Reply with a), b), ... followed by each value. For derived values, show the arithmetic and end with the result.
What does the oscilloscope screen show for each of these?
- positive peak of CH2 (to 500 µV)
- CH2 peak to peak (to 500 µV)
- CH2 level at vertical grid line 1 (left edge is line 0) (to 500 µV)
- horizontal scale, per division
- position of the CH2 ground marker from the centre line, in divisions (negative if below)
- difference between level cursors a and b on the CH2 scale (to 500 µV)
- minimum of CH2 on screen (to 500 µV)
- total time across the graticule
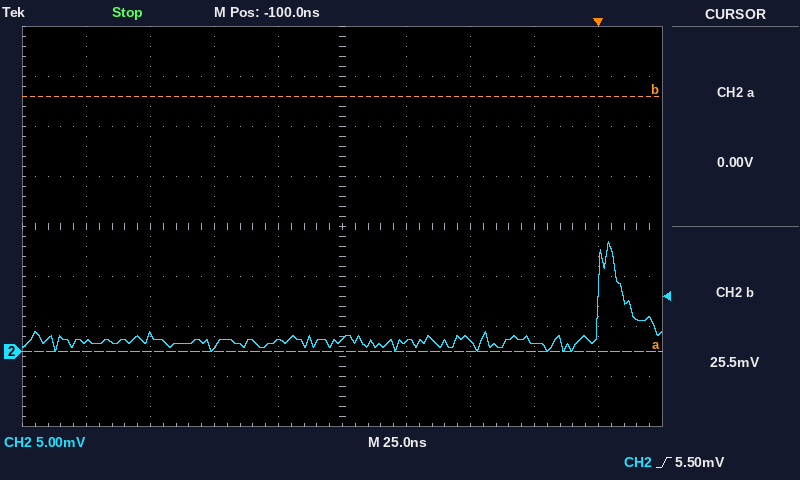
a) 11.0 mV
b) 11.0 mV − (0.0 mV) = 11.0 mV
c) 1.0 mV
d) 25 ns
e) -2.5 div
f) 25.5 mV
g) 0.0 mV
h) 250 ns
